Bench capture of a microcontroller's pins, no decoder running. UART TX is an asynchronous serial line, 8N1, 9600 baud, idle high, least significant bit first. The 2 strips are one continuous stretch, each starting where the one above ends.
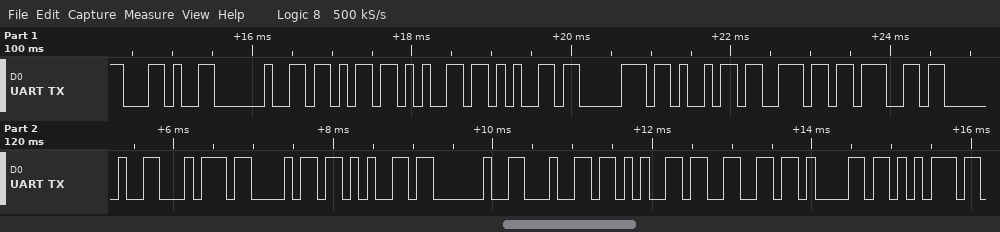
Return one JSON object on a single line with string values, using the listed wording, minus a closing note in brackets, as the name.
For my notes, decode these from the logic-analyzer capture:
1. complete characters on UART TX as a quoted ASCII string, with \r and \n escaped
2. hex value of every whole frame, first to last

{"complete characters on UART TX as a quoted ASCII string, with \\r and \\n escaped": "\", keeping the defau\"", "hex value of every whole frame, first to last": "2C 20 6B 65 65 70 69 6E 67 20 74 68 65 20 64 65 66 61 75"}
